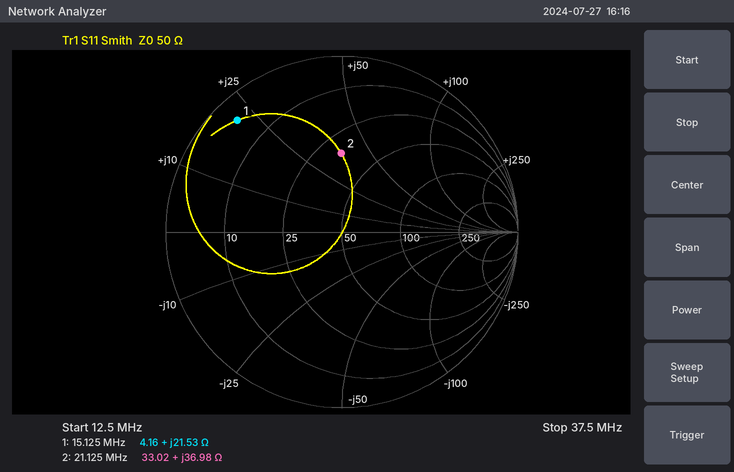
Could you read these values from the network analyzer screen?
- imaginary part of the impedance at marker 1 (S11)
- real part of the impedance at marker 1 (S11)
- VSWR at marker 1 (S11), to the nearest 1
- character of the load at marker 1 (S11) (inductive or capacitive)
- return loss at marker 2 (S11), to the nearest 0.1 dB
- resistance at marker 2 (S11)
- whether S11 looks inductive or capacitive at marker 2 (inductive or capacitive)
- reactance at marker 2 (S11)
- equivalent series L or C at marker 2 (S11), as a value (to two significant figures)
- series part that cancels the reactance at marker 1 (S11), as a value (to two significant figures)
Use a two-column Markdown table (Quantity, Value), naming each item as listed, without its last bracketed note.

| Quantity | Value |
|---|---|
| imaginary part of the impedance at marker 1 | +21.53 Ω |
| real part of the impedance at marker 1 | 4.16 Ω |
| VSWR at marker 1 (S11), to the nearest 1 | 14 |
| character of the load at marker 1 (S11) | inductive |
| return loss at marker 2 (S11), to the nearest 0.1 dB | 7.0 dB |
| resistance at marker 2 | 33.02 Ω |
| whether S11 looks inductive or capacitive at marker 2 | inductive |
| reactance at marker 2 | +36.98 Ω |
| equivalent series L or C at marker 2 (S11), as a value | 280 nH |
| series part that cancels the reactance at marker 1 (S11), as a value | 490 pF |
